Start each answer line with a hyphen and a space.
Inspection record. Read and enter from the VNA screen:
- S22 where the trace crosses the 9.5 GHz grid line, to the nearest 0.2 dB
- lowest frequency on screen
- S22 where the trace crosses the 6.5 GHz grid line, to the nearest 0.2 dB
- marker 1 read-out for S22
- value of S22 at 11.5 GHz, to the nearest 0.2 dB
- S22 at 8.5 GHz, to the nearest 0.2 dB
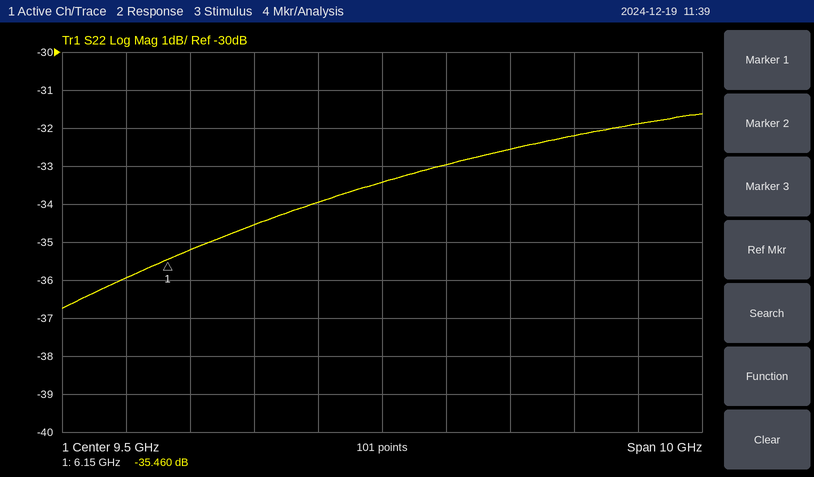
- -33.4 dB
- 4.5 GHz
- -35.2 dB
- -35.460 dB
- -32.6 dB
- -34.0 dB
